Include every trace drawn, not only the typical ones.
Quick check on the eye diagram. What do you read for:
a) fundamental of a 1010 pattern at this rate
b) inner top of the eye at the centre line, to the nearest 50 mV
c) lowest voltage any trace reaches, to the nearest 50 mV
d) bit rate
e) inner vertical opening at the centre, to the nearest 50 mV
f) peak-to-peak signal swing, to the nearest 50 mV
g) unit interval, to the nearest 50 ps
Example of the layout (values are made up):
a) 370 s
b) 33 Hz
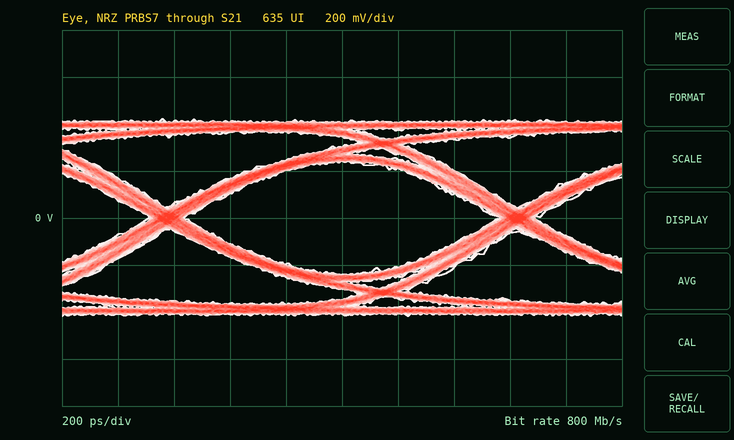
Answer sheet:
a) 400 MHz
b) 250 mV
c) -400 mV
d) 800 Mb/s
e) 500 mV
f) 850 mV
g) 1.25 ns
